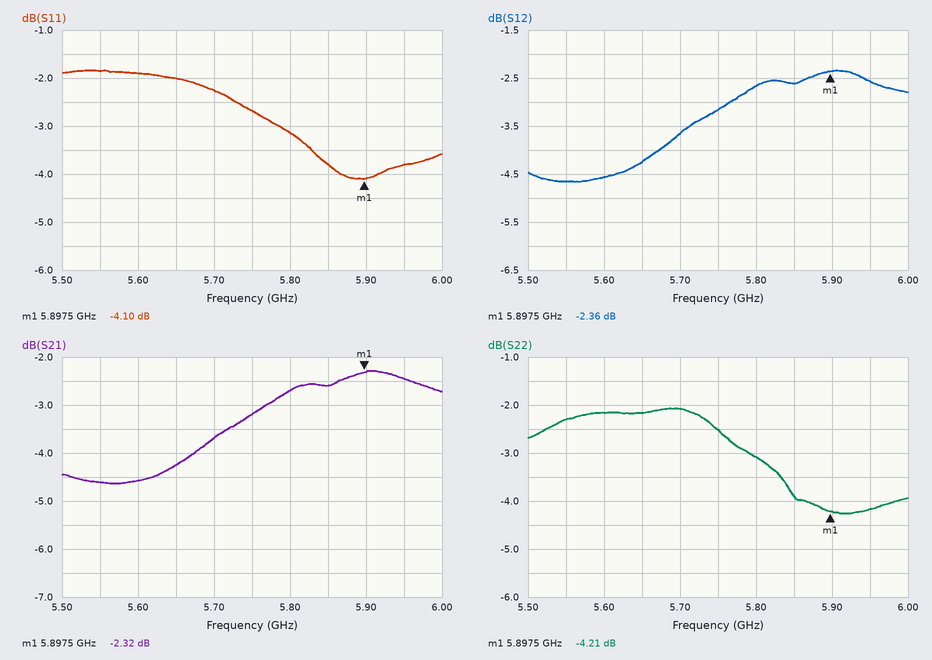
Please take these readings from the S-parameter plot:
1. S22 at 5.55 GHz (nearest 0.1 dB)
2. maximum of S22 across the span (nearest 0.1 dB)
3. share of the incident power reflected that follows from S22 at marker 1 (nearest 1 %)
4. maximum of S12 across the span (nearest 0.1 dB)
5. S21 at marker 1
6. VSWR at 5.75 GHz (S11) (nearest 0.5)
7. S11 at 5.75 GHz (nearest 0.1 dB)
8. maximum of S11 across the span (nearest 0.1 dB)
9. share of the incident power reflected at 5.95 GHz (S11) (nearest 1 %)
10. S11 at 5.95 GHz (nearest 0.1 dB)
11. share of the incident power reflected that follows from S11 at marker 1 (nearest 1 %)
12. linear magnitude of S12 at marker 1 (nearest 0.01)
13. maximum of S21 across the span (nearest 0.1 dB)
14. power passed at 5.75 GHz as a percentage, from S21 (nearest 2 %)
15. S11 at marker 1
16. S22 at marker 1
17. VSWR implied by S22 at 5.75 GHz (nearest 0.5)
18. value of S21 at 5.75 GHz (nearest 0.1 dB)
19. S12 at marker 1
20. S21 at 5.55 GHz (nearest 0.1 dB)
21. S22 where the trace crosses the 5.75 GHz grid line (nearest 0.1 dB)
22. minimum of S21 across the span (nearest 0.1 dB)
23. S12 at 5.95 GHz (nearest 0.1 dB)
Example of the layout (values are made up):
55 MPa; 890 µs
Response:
-2.3 dB; -2.1 dB; 38 %; -2.3 dB; -2.32 dB; 6.5; -2.7 dB; -1.8 dB; 42 %; -3.8 dB; 39 %; 0.76; -2.3 dB; 48 %; -4.10 dB; -4.21 dB; 7.0; -3.2 dB; -2.36 dB; -4.6 dB; -2.5 dB; -4.6 dB; -2.6 dB
